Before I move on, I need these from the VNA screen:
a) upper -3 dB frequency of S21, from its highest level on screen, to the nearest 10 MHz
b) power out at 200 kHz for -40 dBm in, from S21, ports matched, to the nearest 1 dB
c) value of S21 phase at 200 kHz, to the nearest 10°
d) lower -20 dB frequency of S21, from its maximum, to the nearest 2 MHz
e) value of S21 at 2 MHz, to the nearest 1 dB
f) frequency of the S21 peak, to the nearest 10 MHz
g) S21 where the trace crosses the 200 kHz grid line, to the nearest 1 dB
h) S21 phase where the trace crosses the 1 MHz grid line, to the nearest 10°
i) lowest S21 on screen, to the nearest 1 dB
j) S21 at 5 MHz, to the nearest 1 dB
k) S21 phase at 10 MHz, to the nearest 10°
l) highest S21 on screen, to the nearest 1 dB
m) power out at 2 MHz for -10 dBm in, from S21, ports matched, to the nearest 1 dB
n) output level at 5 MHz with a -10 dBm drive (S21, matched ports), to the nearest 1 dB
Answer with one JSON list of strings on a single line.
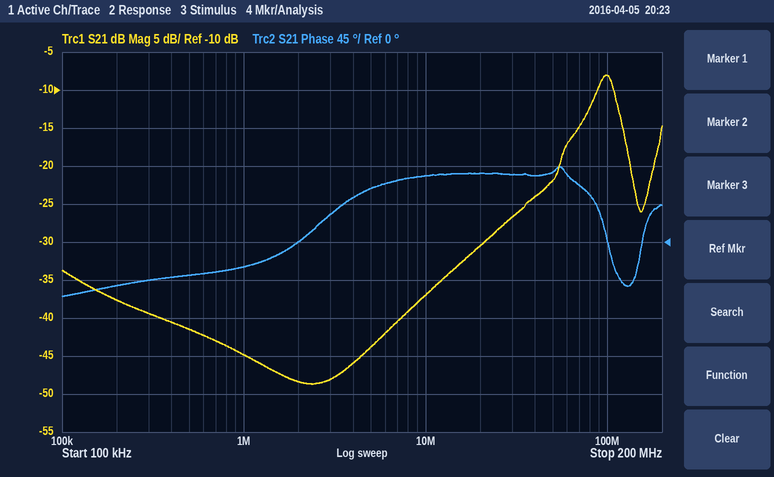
["110 MHz", "-78 dBm", "-50°", "26 MHz", "-48 dB", "100 MHz", "-38 dB", "-30°", "-49 dB", "-44 dB", "80°", "-8 dB", "-58 dBm", "-54 dBm"]
